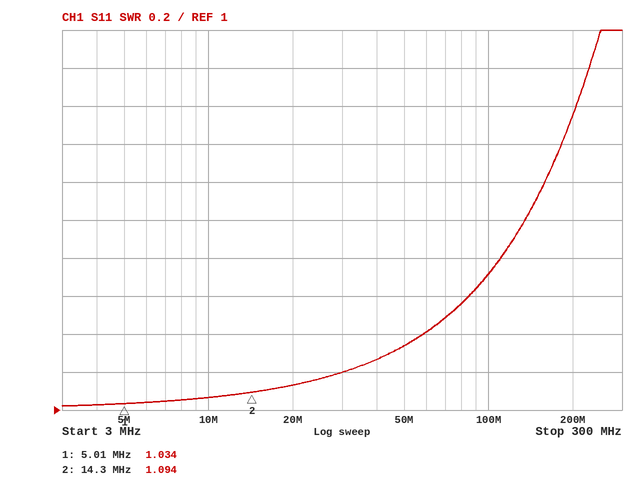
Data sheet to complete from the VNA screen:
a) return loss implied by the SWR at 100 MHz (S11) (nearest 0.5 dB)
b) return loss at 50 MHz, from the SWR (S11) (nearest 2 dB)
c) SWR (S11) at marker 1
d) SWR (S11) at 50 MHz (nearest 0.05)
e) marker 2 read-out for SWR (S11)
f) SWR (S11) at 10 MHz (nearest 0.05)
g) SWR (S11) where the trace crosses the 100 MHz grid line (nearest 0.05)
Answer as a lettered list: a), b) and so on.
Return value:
a) 11.5 dB
b) 16 dB
c) 1.034
d) 1.35
e) 1.094
f) 1.05
g) 1.70
